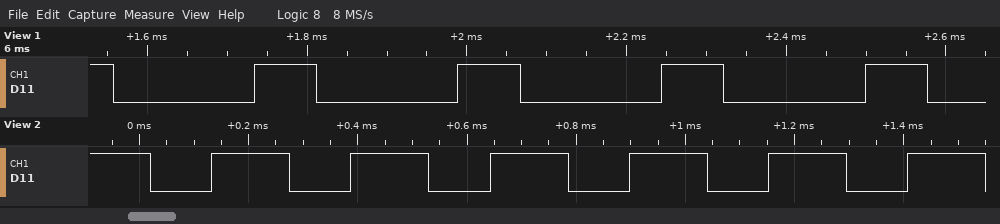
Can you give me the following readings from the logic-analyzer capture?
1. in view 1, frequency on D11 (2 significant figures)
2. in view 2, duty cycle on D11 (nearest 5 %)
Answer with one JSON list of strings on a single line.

["3.9 kHz", "55 %"]
